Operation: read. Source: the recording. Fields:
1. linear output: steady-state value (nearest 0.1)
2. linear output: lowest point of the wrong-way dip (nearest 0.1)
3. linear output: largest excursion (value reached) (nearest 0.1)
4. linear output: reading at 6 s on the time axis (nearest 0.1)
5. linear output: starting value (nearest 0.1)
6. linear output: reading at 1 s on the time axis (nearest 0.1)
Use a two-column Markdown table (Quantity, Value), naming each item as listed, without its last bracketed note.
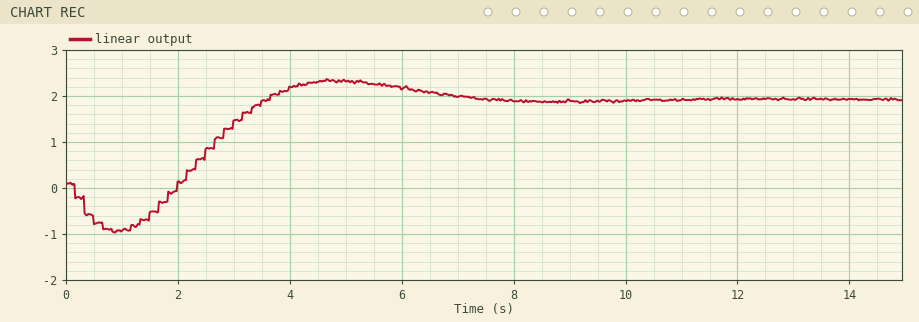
| Quantity | Value |
|---|---|
| linear output: steady-state value | 1.9 |
| linear output: lowest point of the wrong-way dip | -0.9 |
| linear output: largest excursion (value reached) | 2.3 |
| linear output: reading at 6 s on the time axis | 2.2 |
| linear output: starting value | 0.1 |
| linear output: reading at 1 s on the time axis | -0.9 |
